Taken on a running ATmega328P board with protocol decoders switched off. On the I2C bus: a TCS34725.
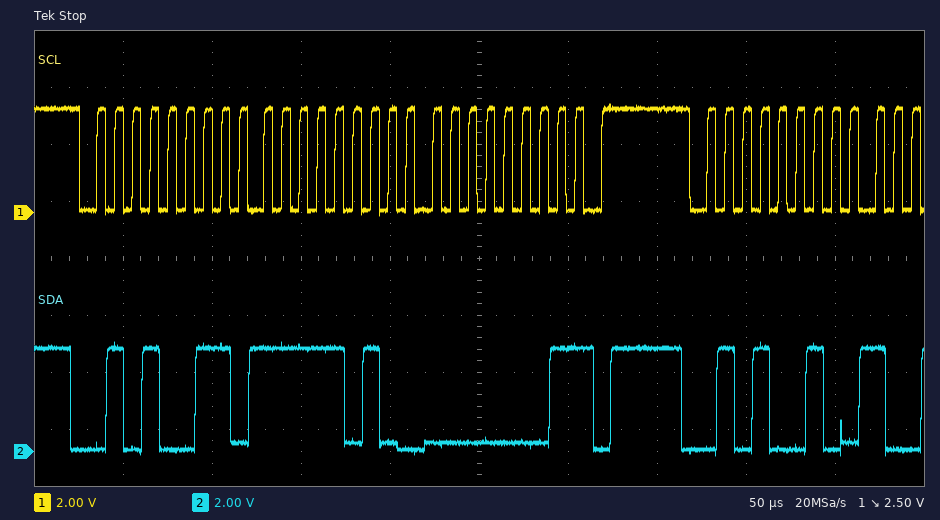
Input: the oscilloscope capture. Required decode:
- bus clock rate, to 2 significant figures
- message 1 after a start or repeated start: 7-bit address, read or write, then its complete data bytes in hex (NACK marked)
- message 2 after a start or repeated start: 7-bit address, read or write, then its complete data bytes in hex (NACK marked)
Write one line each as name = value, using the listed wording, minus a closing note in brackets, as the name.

bus clock rate, to 2 significant figures = 100 kHz
message 1 after a start or repeated start: 7-bit address, read or write, then its complete data bytes in hex = 0x29 read: FA 01 NACK
message 2 after a start or repeated start: 7-bit address, read or write, then its complete data bytes in hex = 0x29 write
